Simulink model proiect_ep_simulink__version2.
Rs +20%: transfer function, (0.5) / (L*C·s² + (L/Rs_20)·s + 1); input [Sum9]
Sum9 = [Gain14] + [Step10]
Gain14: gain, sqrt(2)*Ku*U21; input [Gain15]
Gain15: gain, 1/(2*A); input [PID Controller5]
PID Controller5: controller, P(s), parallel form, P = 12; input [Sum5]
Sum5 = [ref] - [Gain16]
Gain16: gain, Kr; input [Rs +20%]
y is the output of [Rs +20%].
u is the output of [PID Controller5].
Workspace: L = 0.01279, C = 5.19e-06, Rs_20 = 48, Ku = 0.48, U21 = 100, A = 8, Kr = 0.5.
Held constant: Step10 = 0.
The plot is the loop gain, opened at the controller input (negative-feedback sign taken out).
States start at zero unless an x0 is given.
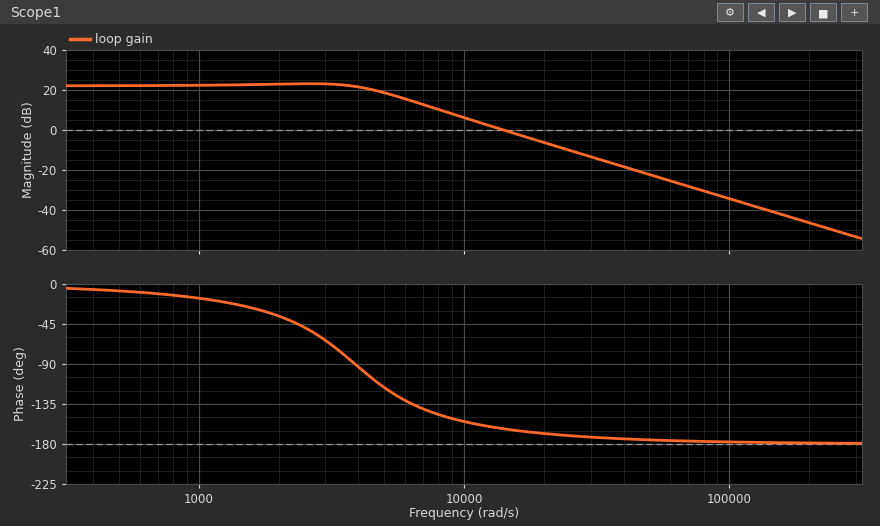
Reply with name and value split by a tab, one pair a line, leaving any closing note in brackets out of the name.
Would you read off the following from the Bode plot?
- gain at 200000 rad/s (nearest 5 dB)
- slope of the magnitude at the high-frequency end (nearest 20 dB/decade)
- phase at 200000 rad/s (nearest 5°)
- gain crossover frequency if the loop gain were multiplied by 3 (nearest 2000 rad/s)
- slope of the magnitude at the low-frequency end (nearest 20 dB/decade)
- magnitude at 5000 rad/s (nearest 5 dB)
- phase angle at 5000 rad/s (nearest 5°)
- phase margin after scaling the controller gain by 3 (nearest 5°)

gain at 200000 rad/s	-45 dB
slope of the magnitude at the high-frequency end	-40 dB/decade
phase at 200000 rad/s	-180°
gain crossover frequency if the loop gain were multiplied by 3	24000 rad/s
slope of the magnitude at the low-frequency end	0 dB/decade
magnitude at 5000 rad/s	20 dB
phase angle at 5000 rad/s	-115°
phase margin after scaling the controller gain by 3	10°
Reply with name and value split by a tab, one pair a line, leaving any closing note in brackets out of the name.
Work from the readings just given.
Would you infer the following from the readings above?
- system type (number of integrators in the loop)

system type	0
